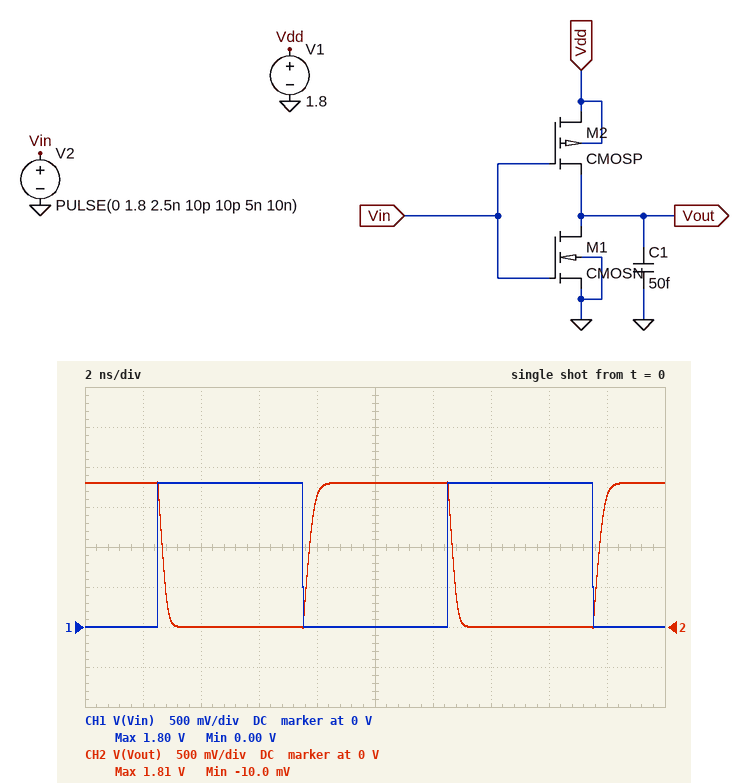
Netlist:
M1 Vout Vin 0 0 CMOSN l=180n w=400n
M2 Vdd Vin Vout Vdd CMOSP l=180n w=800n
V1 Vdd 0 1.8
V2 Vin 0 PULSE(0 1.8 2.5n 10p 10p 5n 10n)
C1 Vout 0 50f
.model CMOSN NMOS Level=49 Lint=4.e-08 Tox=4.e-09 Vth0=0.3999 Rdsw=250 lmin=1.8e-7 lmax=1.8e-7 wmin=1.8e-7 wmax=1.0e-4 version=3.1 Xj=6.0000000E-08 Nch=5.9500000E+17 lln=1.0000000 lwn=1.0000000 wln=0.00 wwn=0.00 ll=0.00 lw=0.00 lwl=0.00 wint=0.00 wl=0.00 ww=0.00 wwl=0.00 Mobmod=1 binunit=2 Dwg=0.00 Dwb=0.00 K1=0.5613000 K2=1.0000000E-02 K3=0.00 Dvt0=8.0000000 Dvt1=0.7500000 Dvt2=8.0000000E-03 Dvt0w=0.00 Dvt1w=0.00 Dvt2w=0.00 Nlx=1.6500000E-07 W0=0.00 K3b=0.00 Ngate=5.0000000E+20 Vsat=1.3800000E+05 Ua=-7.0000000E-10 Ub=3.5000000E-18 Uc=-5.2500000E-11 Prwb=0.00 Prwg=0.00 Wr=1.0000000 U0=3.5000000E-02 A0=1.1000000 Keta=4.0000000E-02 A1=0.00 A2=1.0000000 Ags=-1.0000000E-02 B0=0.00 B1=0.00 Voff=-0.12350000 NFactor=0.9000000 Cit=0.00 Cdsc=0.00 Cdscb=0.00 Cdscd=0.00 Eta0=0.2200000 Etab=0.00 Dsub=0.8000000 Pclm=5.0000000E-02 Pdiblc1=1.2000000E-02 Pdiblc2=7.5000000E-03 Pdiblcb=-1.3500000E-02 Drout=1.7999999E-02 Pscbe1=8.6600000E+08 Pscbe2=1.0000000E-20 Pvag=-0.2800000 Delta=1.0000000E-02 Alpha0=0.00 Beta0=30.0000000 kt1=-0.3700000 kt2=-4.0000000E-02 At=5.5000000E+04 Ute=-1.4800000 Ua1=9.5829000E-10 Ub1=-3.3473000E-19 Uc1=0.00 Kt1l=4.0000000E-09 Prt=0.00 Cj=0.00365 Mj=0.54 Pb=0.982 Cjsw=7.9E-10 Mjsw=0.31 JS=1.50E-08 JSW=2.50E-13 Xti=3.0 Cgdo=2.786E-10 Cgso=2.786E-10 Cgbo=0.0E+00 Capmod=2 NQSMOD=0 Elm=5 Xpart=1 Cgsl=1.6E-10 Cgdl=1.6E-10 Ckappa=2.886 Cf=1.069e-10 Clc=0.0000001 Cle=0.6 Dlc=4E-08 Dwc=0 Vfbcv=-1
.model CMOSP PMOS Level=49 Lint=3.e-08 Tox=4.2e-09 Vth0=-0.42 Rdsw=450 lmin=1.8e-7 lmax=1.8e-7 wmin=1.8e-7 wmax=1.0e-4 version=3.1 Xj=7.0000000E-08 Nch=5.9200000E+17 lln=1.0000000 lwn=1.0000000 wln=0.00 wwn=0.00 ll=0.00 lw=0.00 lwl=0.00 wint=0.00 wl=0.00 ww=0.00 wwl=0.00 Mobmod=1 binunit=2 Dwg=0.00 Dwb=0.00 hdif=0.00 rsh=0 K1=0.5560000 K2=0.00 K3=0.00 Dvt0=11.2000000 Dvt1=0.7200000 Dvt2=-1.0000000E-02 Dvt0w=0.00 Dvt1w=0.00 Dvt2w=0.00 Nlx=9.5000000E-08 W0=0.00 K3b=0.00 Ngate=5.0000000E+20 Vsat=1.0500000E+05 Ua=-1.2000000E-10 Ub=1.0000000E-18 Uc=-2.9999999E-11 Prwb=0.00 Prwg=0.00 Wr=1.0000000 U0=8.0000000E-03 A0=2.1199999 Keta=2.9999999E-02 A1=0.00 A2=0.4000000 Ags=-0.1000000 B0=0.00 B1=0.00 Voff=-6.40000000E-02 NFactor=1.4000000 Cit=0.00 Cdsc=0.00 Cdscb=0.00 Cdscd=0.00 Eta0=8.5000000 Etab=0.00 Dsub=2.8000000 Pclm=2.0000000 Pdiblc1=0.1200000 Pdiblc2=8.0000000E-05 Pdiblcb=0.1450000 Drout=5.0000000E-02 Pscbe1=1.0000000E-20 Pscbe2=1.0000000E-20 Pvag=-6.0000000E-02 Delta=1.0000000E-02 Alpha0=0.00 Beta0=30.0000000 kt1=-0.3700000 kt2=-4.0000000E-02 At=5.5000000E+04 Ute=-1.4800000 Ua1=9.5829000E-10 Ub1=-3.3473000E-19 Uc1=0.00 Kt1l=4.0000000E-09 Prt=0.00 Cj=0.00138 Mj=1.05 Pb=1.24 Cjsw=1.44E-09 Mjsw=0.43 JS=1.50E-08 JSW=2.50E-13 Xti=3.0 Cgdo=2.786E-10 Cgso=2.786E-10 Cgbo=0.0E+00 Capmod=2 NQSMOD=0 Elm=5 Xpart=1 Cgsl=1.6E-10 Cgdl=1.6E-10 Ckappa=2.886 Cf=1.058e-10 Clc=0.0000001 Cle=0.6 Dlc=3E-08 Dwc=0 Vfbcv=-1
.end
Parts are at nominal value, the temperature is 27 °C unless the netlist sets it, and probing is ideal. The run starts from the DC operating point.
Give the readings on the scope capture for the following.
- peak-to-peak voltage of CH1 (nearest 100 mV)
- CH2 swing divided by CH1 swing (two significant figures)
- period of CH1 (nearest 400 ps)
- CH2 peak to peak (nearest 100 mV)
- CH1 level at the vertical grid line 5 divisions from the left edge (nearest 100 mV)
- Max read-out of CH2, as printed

1.8 V
1.0
10.0 ns
1.8 V
0 V
1.81 V
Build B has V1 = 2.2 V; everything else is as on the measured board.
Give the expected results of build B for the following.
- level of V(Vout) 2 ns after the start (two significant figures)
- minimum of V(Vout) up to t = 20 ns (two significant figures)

2.2 V
10 mV
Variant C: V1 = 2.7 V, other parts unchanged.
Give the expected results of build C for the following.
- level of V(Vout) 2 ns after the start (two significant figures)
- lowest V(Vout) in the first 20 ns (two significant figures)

2.7 V
210 mV
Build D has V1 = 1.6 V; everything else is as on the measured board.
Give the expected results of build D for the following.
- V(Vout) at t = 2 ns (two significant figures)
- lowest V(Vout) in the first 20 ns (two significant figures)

1.6 V
-14 mV
